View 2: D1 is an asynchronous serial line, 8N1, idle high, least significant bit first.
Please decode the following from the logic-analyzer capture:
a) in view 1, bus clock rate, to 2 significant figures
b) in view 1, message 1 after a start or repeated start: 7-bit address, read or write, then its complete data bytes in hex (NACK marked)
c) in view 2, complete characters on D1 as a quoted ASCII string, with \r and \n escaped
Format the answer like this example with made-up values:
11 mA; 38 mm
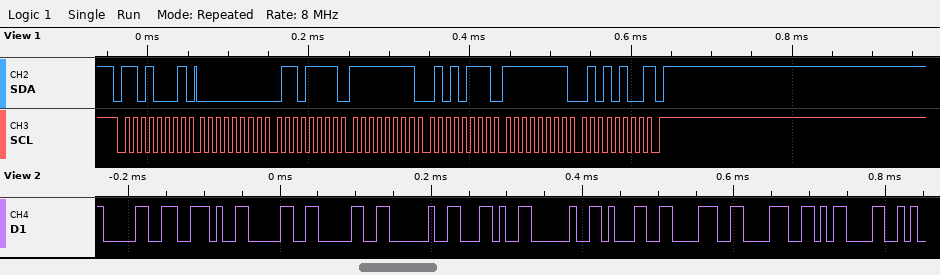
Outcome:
100 kHz; 0x68 read: 00 6F FF 57 FF 54 NACK; "0.00 , 188\r"
